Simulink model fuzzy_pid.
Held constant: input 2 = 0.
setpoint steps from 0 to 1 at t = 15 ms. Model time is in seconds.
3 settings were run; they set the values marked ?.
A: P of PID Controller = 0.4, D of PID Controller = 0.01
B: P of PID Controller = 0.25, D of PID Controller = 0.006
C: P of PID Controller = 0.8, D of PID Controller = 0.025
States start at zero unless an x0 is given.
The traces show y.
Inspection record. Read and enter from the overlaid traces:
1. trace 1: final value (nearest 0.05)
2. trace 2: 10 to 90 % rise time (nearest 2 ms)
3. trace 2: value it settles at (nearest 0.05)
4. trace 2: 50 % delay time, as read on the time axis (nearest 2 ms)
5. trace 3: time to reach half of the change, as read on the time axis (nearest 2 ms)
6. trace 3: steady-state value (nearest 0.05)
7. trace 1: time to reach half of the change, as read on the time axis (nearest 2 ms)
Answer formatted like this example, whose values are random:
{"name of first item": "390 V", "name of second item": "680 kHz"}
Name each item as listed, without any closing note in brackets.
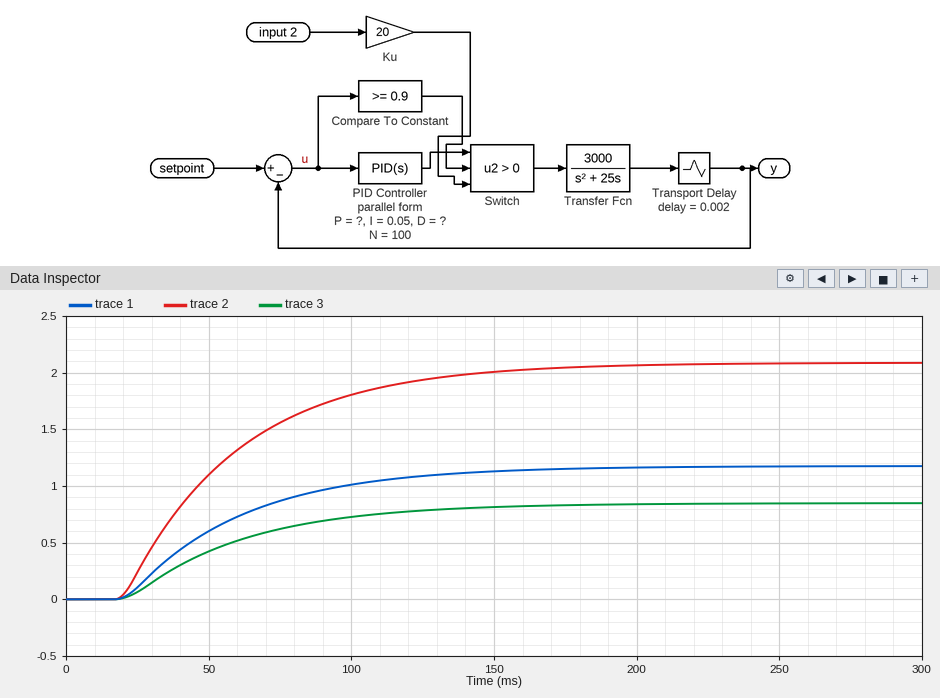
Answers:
{"trace 1: final value": "1.20", "trace 2: 10 to 90 % rise time": "88 ms", "trace 2: value it settles at": "2.10", "trace 2: 50 % delay time, as read on the time axis": "48 ms", "trace 3: time to reach half of the change, as read on the time axis": "50 ms", "trace 3: steady-state value": "0.85", "trace 1: time to reach half of the change, as read on the time axis": "50 ms"}
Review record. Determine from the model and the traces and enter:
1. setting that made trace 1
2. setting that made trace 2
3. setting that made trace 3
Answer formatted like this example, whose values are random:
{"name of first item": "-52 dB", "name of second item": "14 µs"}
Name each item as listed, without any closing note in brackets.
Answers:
{"setting that made trace 1": "A", "setting that made trace 2": "C", "setting that made trace 3": "B"}
